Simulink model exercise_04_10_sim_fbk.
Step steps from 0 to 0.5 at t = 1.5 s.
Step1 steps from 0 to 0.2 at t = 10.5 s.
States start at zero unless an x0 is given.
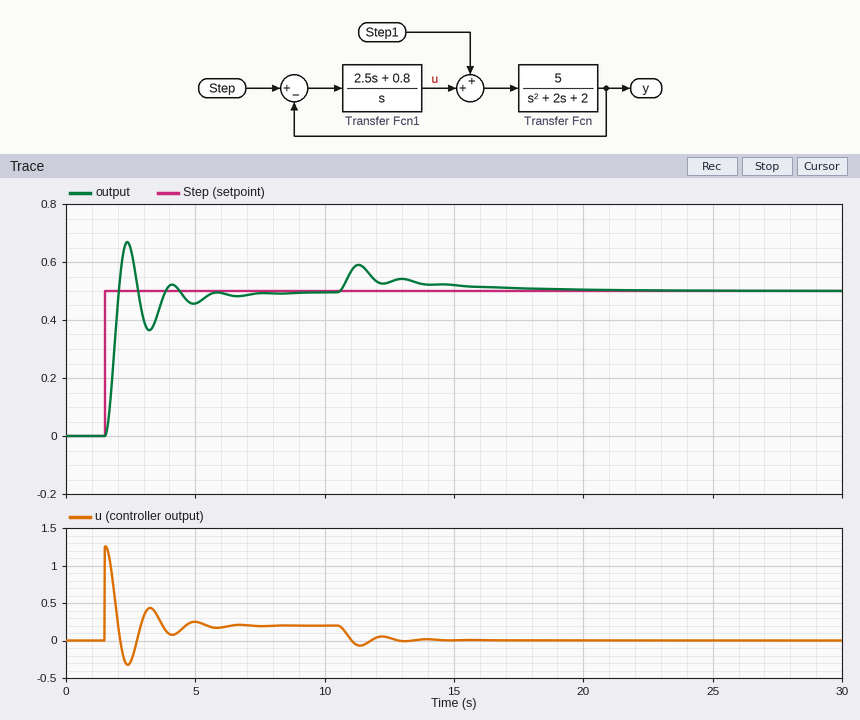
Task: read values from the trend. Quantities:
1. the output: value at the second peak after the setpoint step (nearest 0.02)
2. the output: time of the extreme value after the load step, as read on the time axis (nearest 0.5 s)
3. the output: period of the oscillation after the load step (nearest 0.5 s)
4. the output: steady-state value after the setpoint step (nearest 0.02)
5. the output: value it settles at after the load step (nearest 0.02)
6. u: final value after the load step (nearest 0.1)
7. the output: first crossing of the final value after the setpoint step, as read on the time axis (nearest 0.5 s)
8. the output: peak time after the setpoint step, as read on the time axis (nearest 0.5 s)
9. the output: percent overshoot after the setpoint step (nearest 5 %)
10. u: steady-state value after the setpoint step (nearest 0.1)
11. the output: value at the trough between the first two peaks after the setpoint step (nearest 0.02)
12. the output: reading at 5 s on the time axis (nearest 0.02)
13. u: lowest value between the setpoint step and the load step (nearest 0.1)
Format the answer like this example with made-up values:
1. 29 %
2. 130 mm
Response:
1. 0.52
2. 11.5 s
3. 1.5 s
4. 0.50
5. 0.50
6. 0.0
7. 2.0 s
8. 2.5 s
9. 35 %
10. 0.2
11. 0.36
12. 0.46
13. -0.3
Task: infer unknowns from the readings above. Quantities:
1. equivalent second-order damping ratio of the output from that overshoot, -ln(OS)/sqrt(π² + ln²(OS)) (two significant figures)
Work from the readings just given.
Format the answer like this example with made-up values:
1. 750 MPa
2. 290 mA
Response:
1. 0.32
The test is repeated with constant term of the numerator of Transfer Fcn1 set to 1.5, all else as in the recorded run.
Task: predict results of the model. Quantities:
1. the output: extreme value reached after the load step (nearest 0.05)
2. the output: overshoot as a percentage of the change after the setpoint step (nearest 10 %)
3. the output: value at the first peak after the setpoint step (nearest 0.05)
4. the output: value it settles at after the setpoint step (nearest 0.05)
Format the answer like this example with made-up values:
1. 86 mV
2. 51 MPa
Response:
1. 0.60
2. 40 %
3. 0.70
4. 0.50
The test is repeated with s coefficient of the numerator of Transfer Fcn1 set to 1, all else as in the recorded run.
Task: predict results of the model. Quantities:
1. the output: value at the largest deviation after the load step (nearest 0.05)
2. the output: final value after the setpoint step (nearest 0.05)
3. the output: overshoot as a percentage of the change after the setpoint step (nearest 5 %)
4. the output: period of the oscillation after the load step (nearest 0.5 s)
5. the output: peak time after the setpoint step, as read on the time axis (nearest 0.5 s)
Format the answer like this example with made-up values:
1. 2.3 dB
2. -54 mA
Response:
1. 0.65
2. 0.50
3. 25 %
4. 2.5 s
5. 3.0 s
